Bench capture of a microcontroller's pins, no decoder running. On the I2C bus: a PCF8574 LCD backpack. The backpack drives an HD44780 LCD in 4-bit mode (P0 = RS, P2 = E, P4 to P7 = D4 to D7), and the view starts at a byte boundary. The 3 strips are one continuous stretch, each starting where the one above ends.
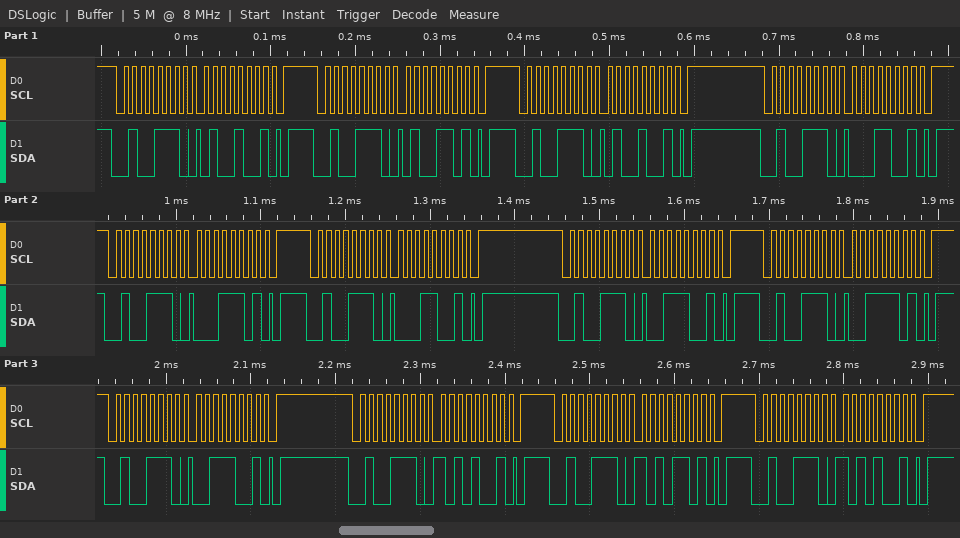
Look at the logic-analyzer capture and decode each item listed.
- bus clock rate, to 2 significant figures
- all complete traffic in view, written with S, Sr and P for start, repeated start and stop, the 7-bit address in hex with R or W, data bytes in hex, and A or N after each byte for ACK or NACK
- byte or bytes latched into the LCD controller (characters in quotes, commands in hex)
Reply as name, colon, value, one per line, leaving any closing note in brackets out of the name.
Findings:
bus clock rate, to 2 significant figures: 100 kHz
all complete traffic in view, written with S, Sr and P for start, repeated start and stop, the 7-bit address in hex with R or W, data bytes in hex, and A or N after each byte for ACK or NACK: S 27W A 49 A P S 27W A 4D A P S 27W A 49 A P S 27W A 19 A P S 27W A 1D A P S 27W A 19 A P S 27W A 39 A P S 27W A 3D A P S 27W A 39 A P S 27W A A9 A P S 27W A AD A P S 27W A A9 A P
byte or bytes latched into the LCD controller: 'A' ':'
